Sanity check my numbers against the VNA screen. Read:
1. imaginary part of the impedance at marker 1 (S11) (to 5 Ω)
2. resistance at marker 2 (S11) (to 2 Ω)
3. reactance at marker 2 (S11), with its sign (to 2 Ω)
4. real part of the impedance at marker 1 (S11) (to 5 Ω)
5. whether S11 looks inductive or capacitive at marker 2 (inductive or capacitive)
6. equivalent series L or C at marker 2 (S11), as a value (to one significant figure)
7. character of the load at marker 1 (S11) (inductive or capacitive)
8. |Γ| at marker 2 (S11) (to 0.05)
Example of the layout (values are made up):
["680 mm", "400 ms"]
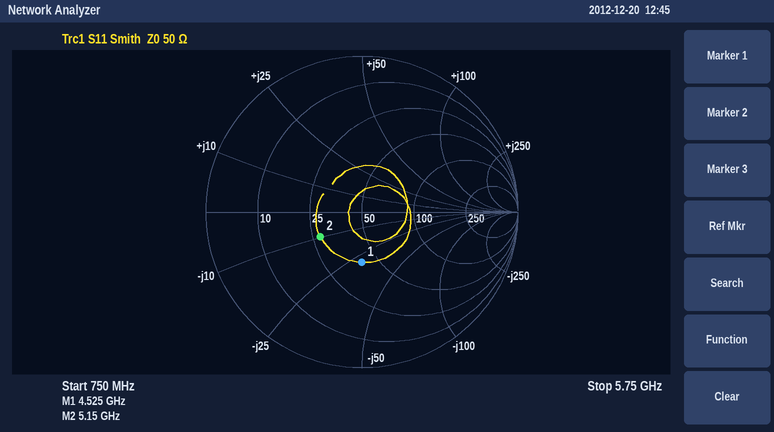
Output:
["-30 Ω", "28 Ω", "-10 Ω", "40 Ω", "capacitive", "3 pF", "capacitive", "0.30"]
